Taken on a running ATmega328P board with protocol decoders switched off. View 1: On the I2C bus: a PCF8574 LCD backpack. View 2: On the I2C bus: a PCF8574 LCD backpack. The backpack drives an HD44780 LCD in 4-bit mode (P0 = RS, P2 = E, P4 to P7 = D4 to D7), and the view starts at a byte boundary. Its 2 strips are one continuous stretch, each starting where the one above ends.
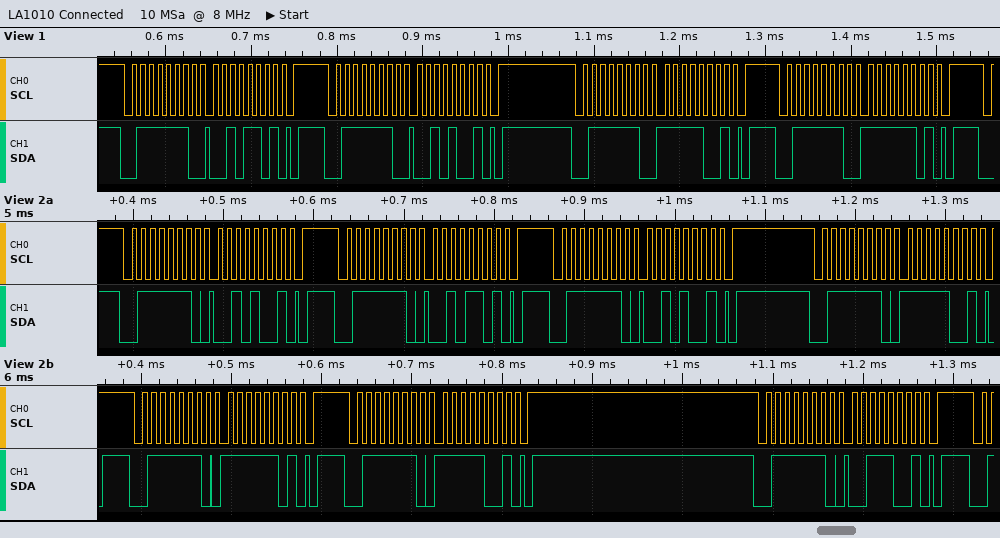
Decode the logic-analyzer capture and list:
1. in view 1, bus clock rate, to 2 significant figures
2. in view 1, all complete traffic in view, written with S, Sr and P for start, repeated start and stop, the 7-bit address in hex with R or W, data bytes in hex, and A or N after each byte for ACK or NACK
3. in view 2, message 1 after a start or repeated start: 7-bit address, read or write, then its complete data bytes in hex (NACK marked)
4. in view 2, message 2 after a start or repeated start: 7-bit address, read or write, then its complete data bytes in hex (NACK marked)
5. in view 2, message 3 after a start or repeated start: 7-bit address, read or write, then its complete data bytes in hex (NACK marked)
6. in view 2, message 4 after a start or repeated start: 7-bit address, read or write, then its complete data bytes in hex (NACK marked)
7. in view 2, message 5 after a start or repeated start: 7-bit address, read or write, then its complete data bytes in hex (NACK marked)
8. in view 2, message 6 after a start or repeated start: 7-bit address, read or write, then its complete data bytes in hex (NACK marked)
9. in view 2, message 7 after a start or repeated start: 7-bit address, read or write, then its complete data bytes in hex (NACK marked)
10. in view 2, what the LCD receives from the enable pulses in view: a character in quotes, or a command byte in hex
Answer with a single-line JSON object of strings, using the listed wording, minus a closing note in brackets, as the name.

{"in view 1, bus clock rate, to 2 significant figures": "100 kHz", "in view 1, all complete traffic in view, written with S, Sr and P for start, repeated start and stop, the 7-bit address in hex with R or W, data bytes in hex, and A or N after each byte for ACK or NACK": "S 3FW A 2D A P S 3FW A 29 A P S 3FW A F9 A P S 3FW A FD A P", "in view 2, message 1 after a start or repeated start: 7-bit address, read or write, then its complete data bytes in hex": "0x3F write: 29", "in view 2, message 2 after a start or repeated start: 7-bit address, read or write, then its complete data bytes in hex": "0x3F write: 2D", "in view 2, message 3 after a start or repeated start: 7-bit address, read or write, then its complete data bytes in hex": "0x3F write: 29", "in view 2, message 4 after a start or repeated start: 7-bit address, read or write, then its complete data bytes in hex": "0x3F write: F9", "in view 2, message 5 after a start or repeated start: 7-bit address, read or write, then its complete data bytes in hex": "0x3F write: FD", "in view 2, message 6 after a start or repeated start: 7-bit address, read or write, then its complete data bytes in hex": "0x3F write: F9", "in view 2, message 7 after a start or repeated start: 7-bit address, read or write, then its complete data bytes in hex": "0x3F write: 39", "in view 2, what the LCD receives from the enable pulses in view: a character in quotes, or a command byte in hex": "'/'"}
